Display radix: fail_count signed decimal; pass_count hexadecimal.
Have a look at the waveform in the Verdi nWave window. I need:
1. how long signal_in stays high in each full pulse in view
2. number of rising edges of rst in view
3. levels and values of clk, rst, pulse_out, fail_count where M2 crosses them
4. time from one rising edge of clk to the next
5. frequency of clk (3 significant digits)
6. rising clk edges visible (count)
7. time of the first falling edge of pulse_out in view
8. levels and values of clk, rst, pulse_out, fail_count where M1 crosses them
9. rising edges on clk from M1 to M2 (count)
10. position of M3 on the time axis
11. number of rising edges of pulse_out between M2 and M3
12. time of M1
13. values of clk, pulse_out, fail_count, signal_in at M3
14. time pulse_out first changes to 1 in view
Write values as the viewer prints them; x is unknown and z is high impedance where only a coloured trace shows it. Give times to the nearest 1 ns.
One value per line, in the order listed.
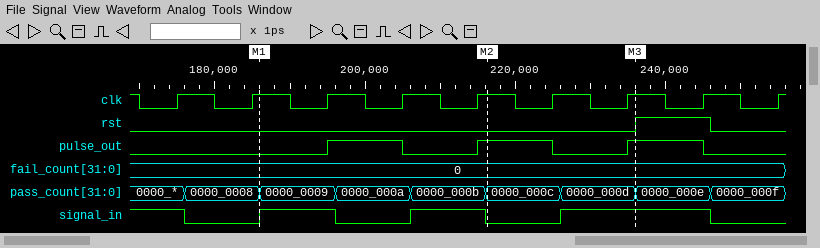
10 ns, 10 ns, 20 ns
1
clk=1, rst=0, pulse_out=1, fail_count=0
10 ns
100 MHz
9
205 ns
clk=1, rst=0, pulse_out=0, fail_count=0
3
236 ns
1
186 ns
clk=1, pulse_out=1, fail_count=0, signal_in=1
195 ns
